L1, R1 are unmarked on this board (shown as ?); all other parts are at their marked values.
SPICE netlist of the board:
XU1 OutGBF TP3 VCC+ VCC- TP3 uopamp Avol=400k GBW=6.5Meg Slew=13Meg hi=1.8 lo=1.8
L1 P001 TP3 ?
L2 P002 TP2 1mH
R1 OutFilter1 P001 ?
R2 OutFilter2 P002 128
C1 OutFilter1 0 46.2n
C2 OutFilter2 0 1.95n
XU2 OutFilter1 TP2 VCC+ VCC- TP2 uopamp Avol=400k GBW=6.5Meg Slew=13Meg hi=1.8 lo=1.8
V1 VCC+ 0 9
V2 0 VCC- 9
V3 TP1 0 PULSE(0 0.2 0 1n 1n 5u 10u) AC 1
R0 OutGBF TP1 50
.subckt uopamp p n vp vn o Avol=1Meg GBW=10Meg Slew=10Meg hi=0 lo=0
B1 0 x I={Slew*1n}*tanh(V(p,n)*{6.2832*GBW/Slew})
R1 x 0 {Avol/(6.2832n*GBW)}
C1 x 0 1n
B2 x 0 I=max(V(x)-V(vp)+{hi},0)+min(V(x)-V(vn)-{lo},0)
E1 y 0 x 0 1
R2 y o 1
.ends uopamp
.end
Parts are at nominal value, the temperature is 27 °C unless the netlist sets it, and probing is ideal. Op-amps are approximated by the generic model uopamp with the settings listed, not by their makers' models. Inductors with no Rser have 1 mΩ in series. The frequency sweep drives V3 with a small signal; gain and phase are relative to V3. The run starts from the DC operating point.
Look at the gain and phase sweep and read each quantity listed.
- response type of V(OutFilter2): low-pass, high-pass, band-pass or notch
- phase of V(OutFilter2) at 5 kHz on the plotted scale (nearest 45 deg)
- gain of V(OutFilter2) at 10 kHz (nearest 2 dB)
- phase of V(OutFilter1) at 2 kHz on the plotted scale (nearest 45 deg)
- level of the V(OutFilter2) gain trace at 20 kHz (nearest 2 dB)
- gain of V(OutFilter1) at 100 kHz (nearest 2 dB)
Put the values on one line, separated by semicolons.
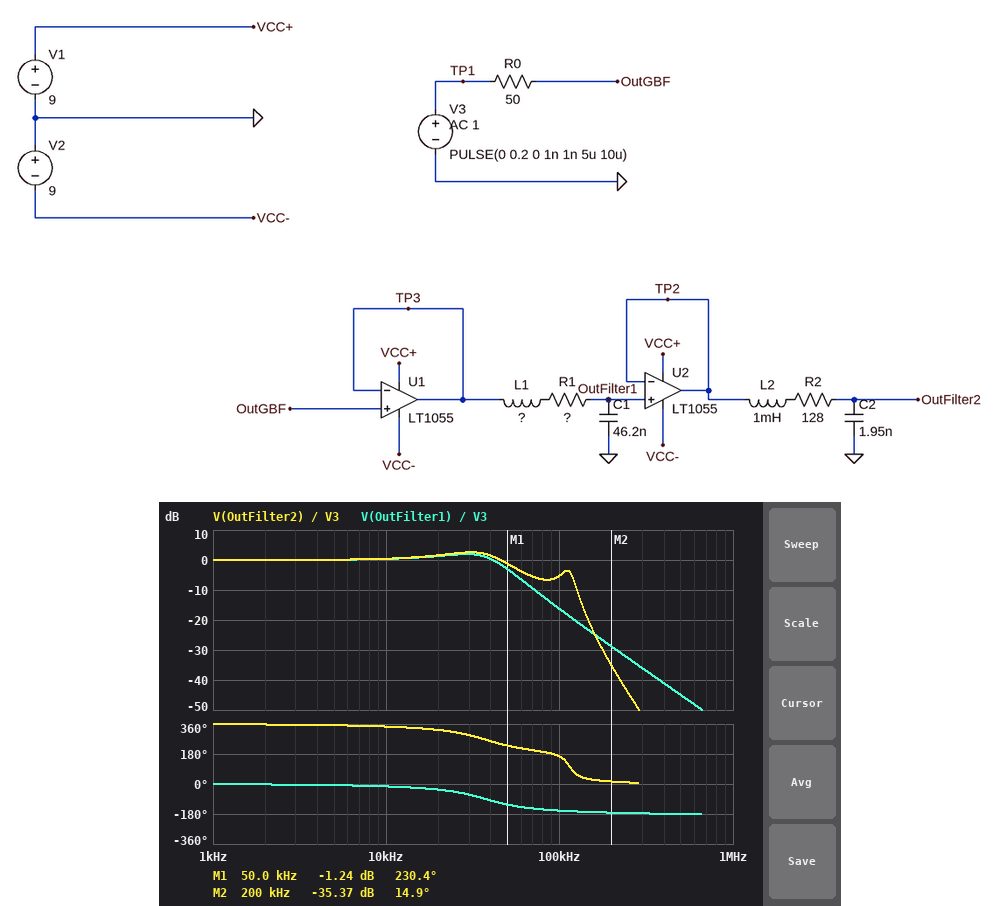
low-pass; 360 deg; 0 dB; 0 deg; 2 dB; -16 dB
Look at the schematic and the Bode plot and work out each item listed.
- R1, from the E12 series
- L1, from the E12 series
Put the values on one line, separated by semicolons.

82 Ω; 390 µH
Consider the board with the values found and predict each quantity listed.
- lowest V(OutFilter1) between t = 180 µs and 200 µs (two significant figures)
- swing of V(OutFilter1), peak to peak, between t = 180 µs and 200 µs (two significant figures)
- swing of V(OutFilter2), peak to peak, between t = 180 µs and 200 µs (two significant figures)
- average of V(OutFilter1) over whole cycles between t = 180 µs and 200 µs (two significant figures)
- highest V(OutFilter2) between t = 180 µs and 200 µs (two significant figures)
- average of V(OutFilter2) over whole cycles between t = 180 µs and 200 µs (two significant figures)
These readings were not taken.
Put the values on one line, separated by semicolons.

81 mV; 38 mV; 140 mV; 100 mV; 170 mV; 100 mV
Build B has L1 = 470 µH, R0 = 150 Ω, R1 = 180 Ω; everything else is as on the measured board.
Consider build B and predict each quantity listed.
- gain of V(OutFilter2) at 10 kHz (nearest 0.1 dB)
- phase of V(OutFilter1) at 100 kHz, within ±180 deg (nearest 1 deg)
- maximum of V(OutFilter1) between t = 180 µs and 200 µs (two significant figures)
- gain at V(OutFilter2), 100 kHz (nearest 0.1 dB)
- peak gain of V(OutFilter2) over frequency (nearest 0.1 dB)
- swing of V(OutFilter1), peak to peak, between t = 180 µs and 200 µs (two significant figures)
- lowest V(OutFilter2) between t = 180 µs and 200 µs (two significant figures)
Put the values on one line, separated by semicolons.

-0.4 dB; -146 deg; 110 mV; -8.2 dB; 0 dB; 28 mV; 50 mV
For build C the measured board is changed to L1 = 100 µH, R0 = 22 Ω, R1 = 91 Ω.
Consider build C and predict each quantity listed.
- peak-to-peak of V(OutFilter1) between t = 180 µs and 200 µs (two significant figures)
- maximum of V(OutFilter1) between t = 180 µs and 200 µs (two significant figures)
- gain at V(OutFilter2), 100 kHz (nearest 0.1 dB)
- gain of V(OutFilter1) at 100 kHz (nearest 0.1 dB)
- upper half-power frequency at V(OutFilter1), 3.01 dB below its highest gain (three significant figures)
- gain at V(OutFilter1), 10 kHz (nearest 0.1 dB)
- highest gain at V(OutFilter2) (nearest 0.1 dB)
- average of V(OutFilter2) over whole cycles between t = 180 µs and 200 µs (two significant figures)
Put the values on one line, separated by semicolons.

98 mV; 150 mV; 2.3 dB; -8.8 dB; 49.2 kHz; -0.1 dB; 4.8 dB; 100 mV
